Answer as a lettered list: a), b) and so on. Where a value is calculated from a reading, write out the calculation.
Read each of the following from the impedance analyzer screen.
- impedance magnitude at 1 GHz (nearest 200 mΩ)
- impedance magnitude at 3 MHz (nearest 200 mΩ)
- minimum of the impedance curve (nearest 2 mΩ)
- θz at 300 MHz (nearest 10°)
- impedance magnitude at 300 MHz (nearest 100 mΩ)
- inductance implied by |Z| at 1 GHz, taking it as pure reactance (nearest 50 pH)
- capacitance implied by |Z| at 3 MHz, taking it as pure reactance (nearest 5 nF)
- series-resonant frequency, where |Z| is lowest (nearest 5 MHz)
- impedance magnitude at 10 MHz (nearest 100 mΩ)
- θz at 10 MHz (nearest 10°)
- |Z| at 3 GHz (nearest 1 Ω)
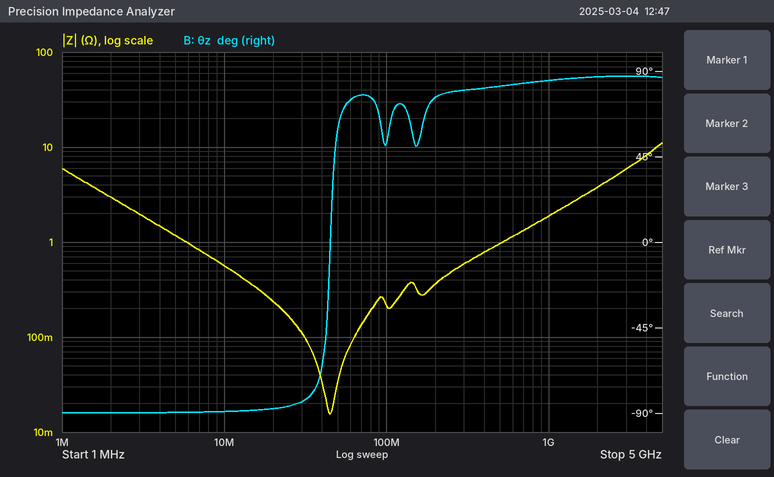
a) 1.8 Ω
b) 2.0 Ω
c) 16 mΩ
d) 80°
e) 600 mΩ
f) L = 1.8 Ω/(2π × 1 GHz) ≈ 286 pH, so 300 pH to the nearest 50 pH
g) C = 1/(2π × 3 MHz × 2.0 Ω) ≈ 26.5 nF, so 25 nF to the nearest 5 nF
h) 45 MHz
i) 600 mΩ
j) -90°
k) 6 Ω
